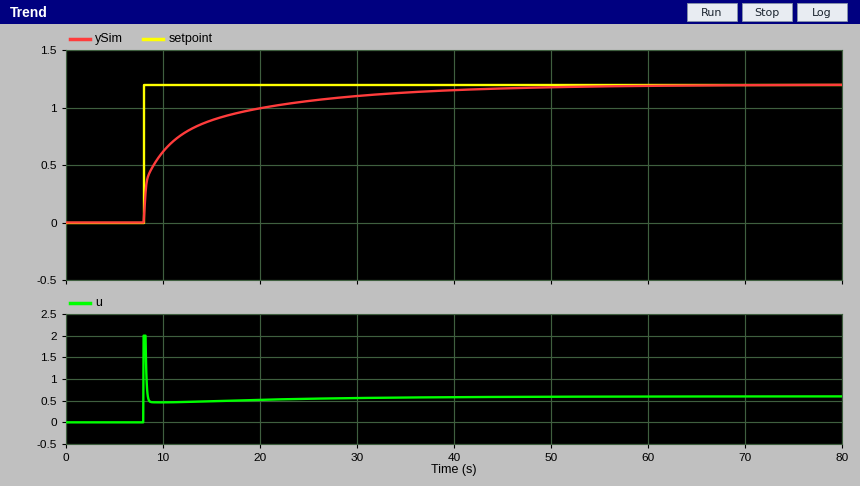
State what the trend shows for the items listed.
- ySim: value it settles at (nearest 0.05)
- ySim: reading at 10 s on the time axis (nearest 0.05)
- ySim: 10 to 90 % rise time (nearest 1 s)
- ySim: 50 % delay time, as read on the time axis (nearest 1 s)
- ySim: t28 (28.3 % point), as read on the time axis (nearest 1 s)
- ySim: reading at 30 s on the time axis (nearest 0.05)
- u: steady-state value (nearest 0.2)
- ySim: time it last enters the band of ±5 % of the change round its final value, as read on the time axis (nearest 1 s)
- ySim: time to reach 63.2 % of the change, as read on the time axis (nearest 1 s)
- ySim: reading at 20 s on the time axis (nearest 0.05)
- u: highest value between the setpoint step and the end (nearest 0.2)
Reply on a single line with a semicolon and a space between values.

1.20; 0.60; 19 s; 10 s; 8 s; 1.10; 0.6; 37 s; 12 s; 1.00; 2.0
